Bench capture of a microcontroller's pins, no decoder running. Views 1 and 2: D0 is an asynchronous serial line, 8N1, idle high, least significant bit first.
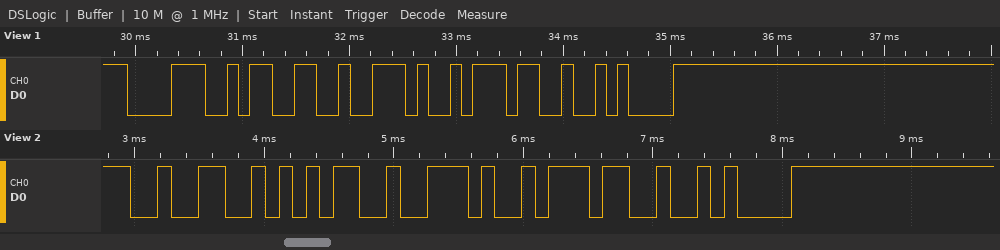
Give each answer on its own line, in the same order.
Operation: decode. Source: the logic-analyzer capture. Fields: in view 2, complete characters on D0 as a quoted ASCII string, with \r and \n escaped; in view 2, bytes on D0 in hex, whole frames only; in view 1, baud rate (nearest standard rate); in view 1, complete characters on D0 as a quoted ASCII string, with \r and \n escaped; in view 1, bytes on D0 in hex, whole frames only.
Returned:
"25.7\n"
32 35 2E 37 0A
9600 baud
"83.7\n"
38 33 2E 37 0A
